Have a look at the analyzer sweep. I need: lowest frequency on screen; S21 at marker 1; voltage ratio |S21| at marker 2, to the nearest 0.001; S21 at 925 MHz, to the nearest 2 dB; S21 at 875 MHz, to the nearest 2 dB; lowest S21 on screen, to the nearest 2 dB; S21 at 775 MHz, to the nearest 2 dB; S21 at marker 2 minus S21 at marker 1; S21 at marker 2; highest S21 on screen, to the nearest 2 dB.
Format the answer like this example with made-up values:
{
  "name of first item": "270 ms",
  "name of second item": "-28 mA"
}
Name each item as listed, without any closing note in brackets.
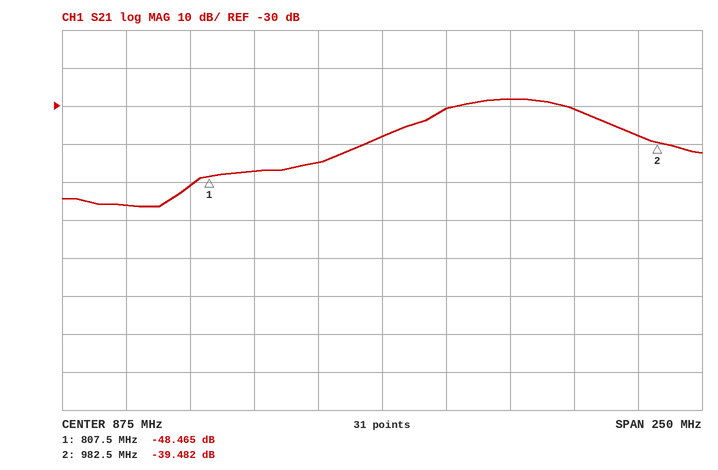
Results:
{
  "lowest frequency on screen": "750 MHz",
  "S21 at marker 1": "-48.465 dB",
  "voltage ratio |S21| at marker 2, to the nearest 0.001": "0.011",
  "S21 at 925 MHz, to the nearest 2 dB": "-28 dB",
  "S21 at 875 MHz, to the nearest 2 dB": "-38 dB",
  "lowest S21 on screen, to the nearest 2 dB": "-56 dB",
  "S21 at 775 MHz, to the nearest 2 dB": "-56 dB",
  "S21 at marker 2 minus S21 at marker 1": "8.983 dB",
  "S21 at marker 2": "-39.482 dB",
  "highest S21 on screen, to the nearest 2 dB": "-28 dB"
}
